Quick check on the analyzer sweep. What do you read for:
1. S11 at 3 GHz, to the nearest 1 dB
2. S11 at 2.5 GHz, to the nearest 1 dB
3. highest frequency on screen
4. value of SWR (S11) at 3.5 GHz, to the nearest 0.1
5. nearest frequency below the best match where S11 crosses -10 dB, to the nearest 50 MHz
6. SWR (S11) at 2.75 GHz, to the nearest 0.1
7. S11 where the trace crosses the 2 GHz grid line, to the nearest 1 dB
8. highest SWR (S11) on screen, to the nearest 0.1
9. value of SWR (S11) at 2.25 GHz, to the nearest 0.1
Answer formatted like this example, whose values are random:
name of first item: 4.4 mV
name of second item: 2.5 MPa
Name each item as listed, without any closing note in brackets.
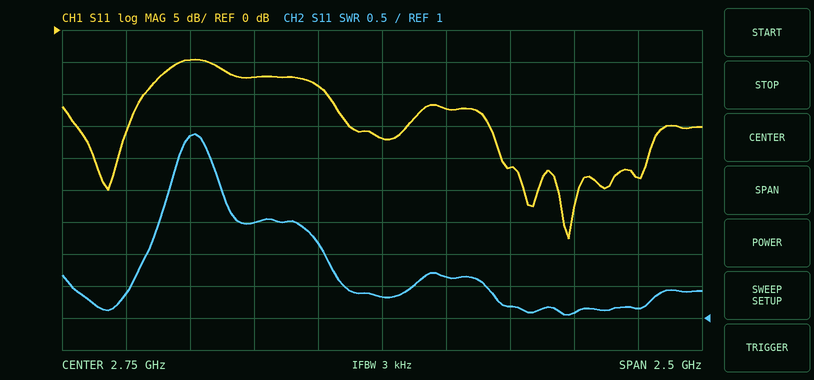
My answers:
S11 at 3 GHz, to the nearest 1 dB: -12 dB
S11 at 2.5 GHz, to the nearest 1 dB: -9 dB
highest frequency on screen: 4 GHz
value of SWR (S11) at 3.5 GHz, to the nearest 0.1: 1.1
nearest frequency below the best match where S11 crosses -10 dB, to the nearest 50 MHz: 2.55 GHz
SWR (S11) at 2.75 GHz, to the nearest 0.1: 1.3
S11 where the trace crosses the 2 GHz grid line, to the nearest 1 dB: -5 dB
highest SWR (S11) on screen, to the nearest 0.1: 3.9
value of SWR (S11) at 2.25 GHz, to the nearest 0.1: 2.5
